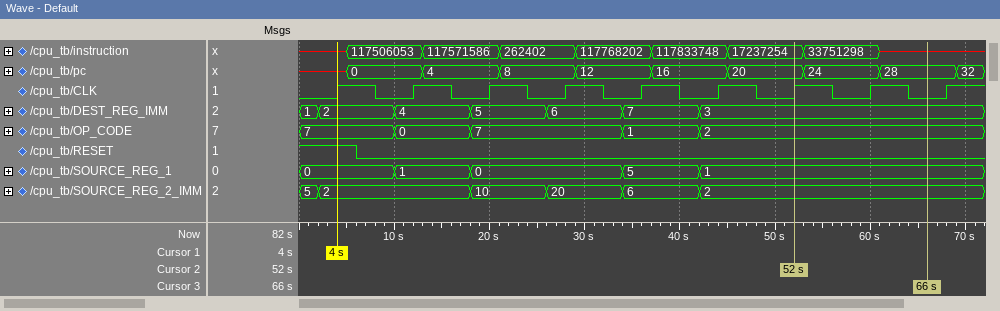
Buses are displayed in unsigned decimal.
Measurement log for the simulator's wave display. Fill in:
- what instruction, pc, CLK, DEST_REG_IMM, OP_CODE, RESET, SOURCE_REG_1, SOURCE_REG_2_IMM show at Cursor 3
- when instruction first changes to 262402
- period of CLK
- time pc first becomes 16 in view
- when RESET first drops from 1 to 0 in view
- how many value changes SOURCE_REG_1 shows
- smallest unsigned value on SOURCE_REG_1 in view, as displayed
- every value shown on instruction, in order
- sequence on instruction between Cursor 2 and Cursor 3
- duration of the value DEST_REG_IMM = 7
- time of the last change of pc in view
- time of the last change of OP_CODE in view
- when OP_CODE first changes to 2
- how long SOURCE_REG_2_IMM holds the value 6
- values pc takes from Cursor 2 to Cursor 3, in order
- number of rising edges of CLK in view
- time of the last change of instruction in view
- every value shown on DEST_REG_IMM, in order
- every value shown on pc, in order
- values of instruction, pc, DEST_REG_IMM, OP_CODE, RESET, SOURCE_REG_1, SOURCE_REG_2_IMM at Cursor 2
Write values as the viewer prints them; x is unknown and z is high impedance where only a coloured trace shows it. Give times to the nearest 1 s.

instruction=x, pc=28, CLK=0, DEST_REG_IMM=3, OP_CODE=2, RESET=0, SOURCE_REG_1=1, SOURCE_REG_2_IMM=2
21 s
8 s
37 s
6 s
4
0
x, 117506053, 117571586, 262402, 117768202, 117833748, 17237254, 33751298, x
17237254, 33751298, x
8 s
69 s
42 s
42 s
8 s
20, 24, 28
9
61 s
1, 2, 4, 5, 6, 7, 3
x, 0, 4, 8, 12, 16, 20, 24, 28, 32
instruction=17237254, pc=20, DEST_REG_IMM=3, OP_CODE=2, RESET=0, SOURCE_REG_1=1, SOURCE_REG_2_IMM=2
